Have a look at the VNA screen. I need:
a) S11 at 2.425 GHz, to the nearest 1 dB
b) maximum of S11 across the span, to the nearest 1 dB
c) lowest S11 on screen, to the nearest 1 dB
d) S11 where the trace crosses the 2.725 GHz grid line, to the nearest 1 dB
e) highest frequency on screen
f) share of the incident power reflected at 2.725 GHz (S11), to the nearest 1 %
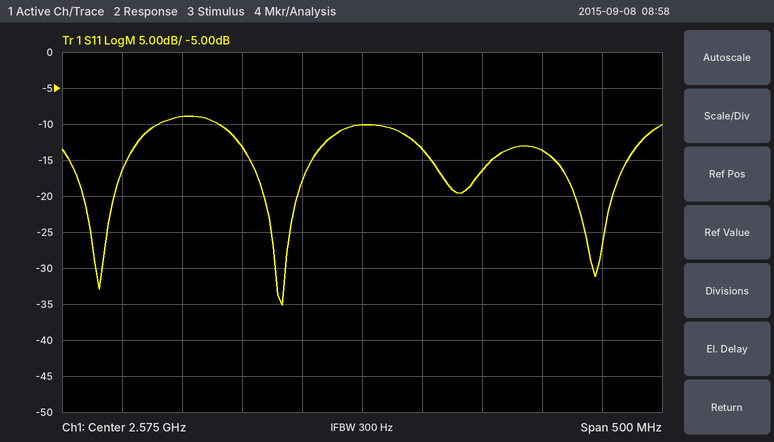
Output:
-9 dB
-9 dB
-35 dB
-14 dB
2.825 GHz
4 %
